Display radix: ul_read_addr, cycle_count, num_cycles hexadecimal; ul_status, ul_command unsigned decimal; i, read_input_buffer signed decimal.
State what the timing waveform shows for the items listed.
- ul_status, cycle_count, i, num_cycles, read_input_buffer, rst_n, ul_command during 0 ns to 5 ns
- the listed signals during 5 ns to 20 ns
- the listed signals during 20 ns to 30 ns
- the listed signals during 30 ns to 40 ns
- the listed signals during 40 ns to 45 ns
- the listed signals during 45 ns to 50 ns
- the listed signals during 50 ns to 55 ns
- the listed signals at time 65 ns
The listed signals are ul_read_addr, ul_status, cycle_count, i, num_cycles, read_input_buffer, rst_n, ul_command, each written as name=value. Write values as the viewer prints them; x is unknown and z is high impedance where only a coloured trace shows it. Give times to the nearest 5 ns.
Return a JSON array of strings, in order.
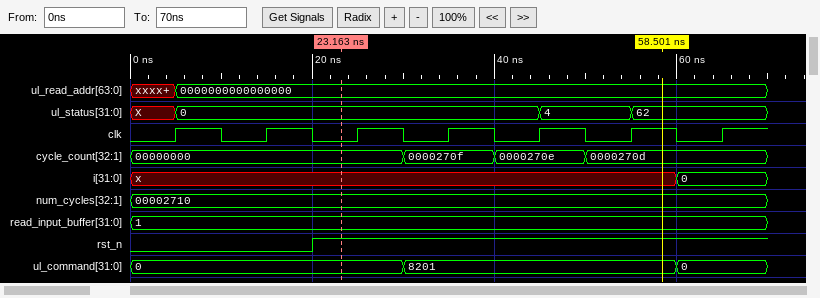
["ul_status=X, cycle_count=00000000, i=x, num_cycles=00002710, read_input_buffer=1, rst_n=0, ul_command=0", "ul_read_addr=0000000000000000, ul_status=0, cycle_count=00000000, i=x, num_cycles=00002710, read_input_buffer=1, rst_n=0, ul_command=0", "ul_read_addr=0000000000000000, ul_status=0, cycle_count=00000000, i=x, num_cycles=00002710, read_input_buffer=1, rst_n=1, ul_command=0", "ul_read_addr=0000000000000000, ul_status=0, cycle_count=0000270f, i=x, num_cycles=00002710, read_input_buffer=1, rst_n=1, ul_command=8201", "ul_read_addr=0000000000000000, ul_status=0, cycle_count=0000270e, i=x, num_cycles=00002710, read_input_buffer=1, rst_n=1, ul_command=8201", "ul_read_addr=0000000000000000, ul_status=4, cycle_count=0000270e, i=x, num_cycles=00002710, read_input_buffer=1, rst_n=1, ul_command=8201", "ul_read_addr=0000000000000000, ul_status=4, cycle_count=0000270d, i=x, num_cycles=00002710, read_input_buffer=1, rst_n=1, ul_command=8201", "ul_read_addr=0000000000000000, ul_status=62, cycle_count=0000270d, i=0, num_cycles=00002710, read_input_buffer=1, rst_n=1, ul_command=0"]
